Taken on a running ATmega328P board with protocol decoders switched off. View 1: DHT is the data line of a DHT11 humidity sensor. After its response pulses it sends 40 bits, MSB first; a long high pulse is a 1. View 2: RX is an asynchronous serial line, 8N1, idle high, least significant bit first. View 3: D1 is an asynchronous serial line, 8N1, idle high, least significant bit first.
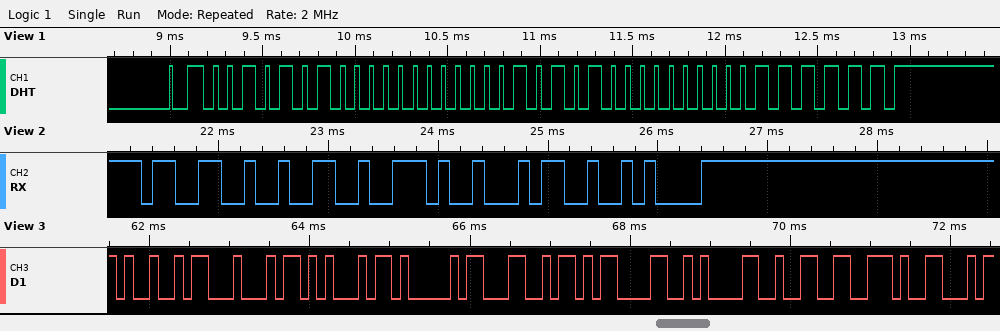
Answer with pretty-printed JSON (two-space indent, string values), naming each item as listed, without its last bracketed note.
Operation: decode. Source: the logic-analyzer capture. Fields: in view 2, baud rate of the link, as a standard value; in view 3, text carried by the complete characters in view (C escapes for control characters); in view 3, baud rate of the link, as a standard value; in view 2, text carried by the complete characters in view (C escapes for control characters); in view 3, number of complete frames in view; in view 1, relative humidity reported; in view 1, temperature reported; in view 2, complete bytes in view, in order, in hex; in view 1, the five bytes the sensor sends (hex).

{
  "in view 2, baud rate of the link, as a standard value": "9600 baud",
  "in view 3, text carried by the complete characters in view": "\"IDEAL\\r\\n2.\"",
  "in view 3, baud rate of the link, as a standard value": "9600 baud",
  "in view 2, text carried by the complete characters in view": "\"32.4\\n\"",
  "in view 3, number of complete frames in view": "9",
  "in view 1, relative humidity reported": "42 %",
  "in view 1, temperature reported": "21.0 °C",
  "in view 2, complete bytes in view, in order, in hex": "33 32 2E 34 0A",
  "in view 1, the five bytes the sensor sends": "2A 00 15 00 3F"
}
